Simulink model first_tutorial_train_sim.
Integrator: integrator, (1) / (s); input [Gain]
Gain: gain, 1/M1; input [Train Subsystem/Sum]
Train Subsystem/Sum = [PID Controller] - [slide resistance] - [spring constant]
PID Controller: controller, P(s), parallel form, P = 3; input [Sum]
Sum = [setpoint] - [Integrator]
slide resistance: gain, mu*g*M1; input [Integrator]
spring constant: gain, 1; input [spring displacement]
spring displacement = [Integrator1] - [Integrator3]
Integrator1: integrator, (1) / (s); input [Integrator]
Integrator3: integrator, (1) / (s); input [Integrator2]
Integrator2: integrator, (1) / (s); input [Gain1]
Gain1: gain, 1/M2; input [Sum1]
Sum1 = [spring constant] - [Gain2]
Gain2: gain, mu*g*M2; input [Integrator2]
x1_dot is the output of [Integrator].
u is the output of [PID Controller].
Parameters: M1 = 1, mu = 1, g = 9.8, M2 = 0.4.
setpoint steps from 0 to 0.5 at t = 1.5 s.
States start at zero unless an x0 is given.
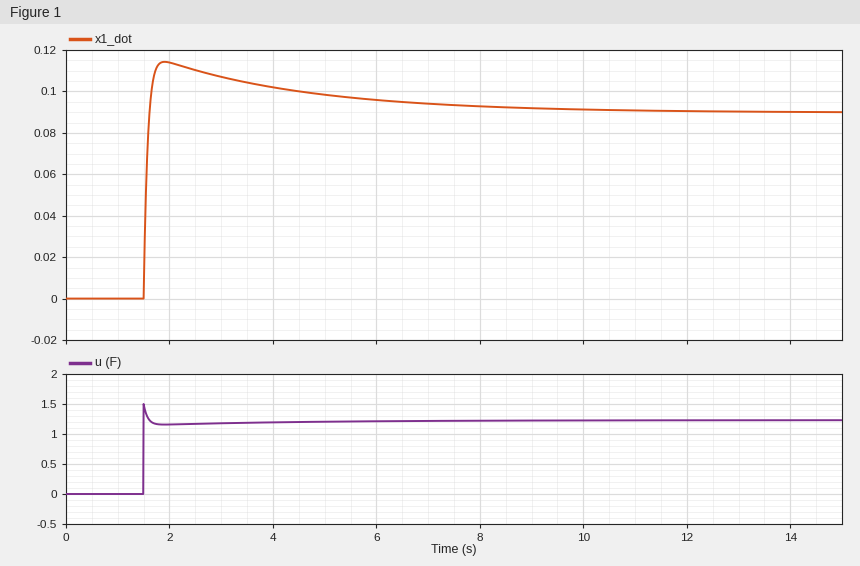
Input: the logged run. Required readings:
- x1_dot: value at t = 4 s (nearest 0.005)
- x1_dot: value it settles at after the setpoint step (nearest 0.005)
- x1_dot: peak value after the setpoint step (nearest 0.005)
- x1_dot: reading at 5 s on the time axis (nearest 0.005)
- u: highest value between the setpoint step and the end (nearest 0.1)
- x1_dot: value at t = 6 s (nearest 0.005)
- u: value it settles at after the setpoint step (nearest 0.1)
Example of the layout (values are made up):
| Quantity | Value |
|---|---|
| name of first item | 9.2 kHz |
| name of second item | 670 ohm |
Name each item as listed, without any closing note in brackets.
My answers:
| Quantity | Value |
|---|---|
| x1_dot: value at t = 4 s | 0.100 |
| x1_dot: value it settles at after the setpoint step | 0.090 |
| x1_dot: peak value after the setpoint step | 0.115 |
| x1_dot: reading at 5 s on the time axis | 0.100 |
| u: highest value between the setpoint step and the end | 1.5 |
| x1_dot: value at t = 6 s | 0.095 |
| u: value it settles at after the setpoint step | 1.2 |
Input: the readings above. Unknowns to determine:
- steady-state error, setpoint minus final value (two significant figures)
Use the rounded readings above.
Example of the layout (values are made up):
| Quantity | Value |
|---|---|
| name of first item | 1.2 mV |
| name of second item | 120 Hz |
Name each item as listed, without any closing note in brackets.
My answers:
| Quantity | Value |
|---|---|
| steady-state error, setpoint minus final value | 0.41 |
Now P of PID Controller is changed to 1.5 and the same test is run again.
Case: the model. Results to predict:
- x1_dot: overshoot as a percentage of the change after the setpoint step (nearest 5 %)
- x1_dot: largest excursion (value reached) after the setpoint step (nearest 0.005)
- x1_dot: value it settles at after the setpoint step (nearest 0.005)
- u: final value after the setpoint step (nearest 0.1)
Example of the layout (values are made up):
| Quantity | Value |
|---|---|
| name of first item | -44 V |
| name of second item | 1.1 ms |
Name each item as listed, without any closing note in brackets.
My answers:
| Quantity | Value |
|---|---|
| x1_dot: overshoot as a percentage of the change after the setpoint step | 30 % |
| x1_dot: largest excursion (value reached) after the setpoint step | 0.065 |
| x1_dot: value it settles at after the setpoint step | 0.050 |
| u: final value after the setpoint step | 0.7 |
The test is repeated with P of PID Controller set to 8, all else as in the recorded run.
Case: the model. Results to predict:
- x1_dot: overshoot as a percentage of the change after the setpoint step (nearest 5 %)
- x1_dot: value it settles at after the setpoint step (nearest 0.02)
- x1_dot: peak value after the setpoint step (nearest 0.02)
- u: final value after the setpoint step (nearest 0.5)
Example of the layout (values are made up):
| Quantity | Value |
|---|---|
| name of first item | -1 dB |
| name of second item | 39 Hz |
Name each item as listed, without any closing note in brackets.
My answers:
| Quantity | Value |
|---|---|
| x1_dot: overshoot as a percentage of the change after the setpoint step | 20 % |
| x1_dot: value it settles at after the setpoint step | 0.18 |
| x1_dot: peak value after the setpoint step | 0.22 |
| u: final value after the setpoint step | 2.5 |
